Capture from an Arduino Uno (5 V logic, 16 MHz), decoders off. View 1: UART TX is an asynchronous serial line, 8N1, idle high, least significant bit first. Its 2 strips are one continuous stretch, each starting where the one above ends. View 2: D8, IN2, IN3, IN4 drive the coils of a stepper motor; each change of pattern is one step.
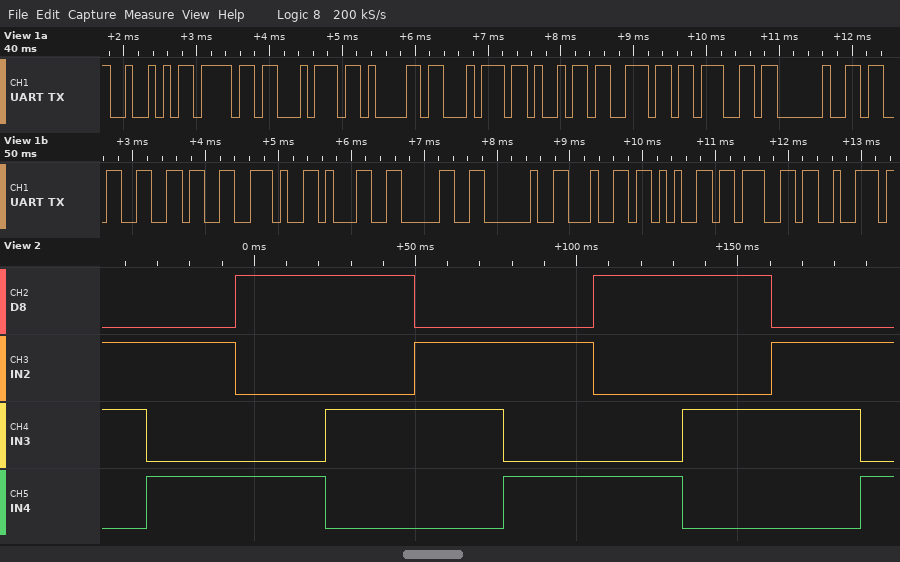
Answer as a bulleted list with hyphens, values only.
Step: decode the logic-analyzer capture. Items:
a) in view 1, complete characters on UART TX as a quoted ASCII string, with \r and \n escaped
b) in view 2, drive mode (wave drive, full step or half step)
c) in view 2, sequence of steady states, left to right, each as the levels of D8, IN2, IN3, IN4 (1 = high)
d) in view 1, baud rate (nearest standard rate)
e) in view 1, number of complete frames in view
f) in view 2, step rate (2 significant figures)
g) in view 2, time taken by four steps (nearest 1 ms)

- "Rotating 36.10 degr"
- full step
- 0110 0101 1001 1010 0110 0101 1001 1010 0110 0101
- 9600 baud
- 19
- 36 steps/s
- 111 ms
